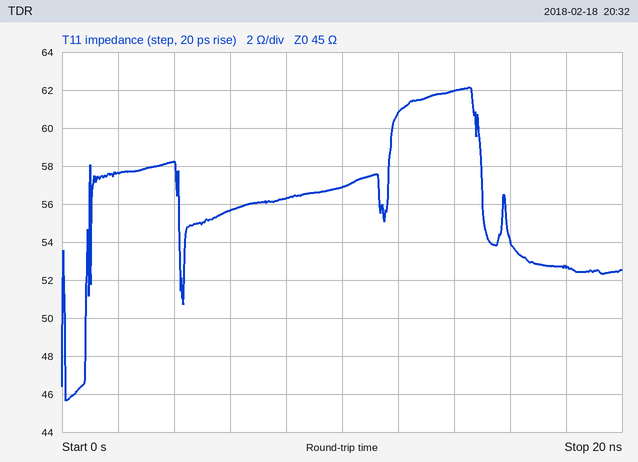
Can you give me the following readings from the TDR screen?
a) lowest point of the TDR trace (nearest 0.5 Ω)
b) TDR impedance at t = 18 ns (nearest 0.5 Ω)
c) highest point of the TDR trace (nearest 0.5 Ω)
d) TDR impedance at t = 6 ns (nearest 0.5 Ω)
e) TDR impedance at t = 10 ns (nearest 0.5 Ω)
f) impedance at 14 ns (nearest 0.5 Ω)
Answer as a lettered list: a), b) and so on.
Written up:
a) 45.5 Ω
b) 52.5 Ω
c) 62.0 Ω
d) 55.5 Ω
e) 57.0 Ω
f) 62.0 Ω
